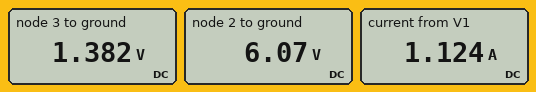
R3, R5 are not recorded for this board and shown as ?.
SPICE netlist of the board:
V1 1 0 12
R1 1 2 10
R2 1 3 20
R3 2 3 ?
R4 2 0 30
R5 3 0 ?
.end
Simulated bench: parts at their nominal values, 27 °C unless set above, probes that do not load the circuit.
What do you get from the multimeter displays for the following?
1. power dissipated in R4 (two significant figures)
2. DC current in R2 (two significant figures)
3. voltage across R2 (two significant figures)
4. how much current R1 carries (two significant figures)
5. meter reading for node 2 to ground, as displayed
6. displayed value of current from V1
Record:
1.2 W
530 mA
11 V
590 mA
6.07 V
1.124 A
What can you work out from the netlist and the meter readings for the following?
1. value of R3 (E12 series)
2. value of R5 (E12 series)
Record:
12 Ω
1.5 Ω
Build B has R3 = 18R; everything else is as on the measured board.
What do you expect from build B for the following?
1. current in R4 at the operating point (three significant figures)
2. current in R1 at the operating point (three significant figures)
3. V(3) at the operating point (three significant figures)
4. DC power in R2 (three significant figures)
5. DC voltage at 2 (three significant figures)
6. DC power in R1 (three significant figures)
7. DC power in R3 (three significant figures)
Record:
224 mA
528 mA
1.26 V
5.77 W
6.72 V
2.78 W
1.66 W
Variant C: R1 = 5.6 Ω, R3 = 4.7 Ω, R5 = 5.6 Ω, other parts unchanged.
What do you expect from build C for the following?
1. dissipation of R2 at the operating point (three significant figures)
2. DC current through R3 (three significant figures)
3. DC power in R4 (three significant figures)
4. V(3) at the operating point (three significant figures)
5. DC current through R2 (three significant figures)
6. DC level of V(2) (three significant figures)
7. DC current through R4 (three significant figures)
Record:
2.45 W
543 mA
1.90 W
5.00 V
350 mA
7.55 V
252 mA
